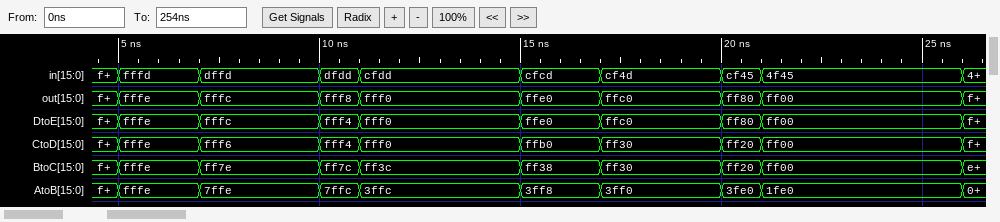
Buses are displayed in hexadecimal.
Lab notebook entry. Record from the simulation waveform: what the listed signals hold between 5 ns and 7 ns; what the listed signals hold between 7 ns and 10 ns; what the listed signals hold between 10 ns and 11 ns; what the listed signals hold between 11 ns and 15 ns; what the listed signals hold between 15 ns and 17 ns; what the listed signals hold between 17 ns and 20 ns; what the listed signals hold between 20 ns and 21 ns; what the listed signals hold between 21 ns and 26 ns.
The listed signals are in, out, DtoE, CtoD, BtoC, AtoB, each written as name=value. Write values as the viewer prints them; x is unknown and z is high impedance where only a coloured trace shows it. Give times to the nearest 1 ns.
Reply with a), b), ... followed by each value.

a) in=fffd, out=fffe, DtoE=fffe, CtoD=fffe, BtoC=fffe, AtoB=fffe
b) in=dffd, out=fffc, DtoE=fffc, CtoD=fff6, BtoC=ff7e, AtoB=7ffe
c) in=dfdd, out=fff8, DtoE=fff4, CtoD=fff4, BtoC=ff7c, AtoB=7ffc
d) in=cfdd, out=fff0, DtoE=fff0, CtoD=fff0, BtoC=ff3c, AtoB=3ffc
e) in=cfcd, out=ffe0, DtoE=ffe0, CtoD=ffb0, BtoC=ff38, AtoB=3ff8
f) in=cf4d, out=ffc0, DtoE=ffc0, CtoD=ff30, BtoC=ff30, AtoB=3ff0
g) in=cf45, out=ff80, DtoE=ff80, CtoD=ff20, BtoC=ff20, AtoB=3fe0
h) in=4f45, out=ff00, DtoE=ff00, CtoD=ff00, BtoC=ff00, AtoB=1fe0
